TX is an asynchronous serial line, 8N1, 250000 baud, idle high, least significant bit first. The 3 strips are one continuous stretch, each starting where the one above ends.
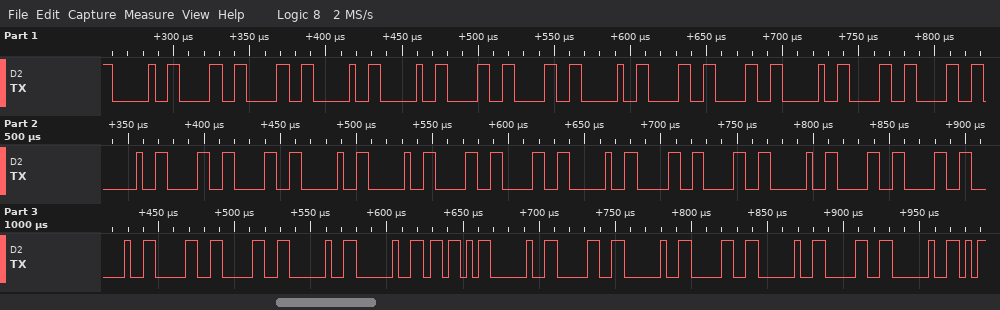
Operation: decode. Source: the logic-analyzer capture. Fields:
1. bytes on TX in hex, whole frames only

20 30 30 20 20 30 30 20 30 30 20 30 30 20 30 30 20 20 30 30 20 30 30 20 30 30 20 30 30 20 20 5B 20 30 20 30 20 30 20
